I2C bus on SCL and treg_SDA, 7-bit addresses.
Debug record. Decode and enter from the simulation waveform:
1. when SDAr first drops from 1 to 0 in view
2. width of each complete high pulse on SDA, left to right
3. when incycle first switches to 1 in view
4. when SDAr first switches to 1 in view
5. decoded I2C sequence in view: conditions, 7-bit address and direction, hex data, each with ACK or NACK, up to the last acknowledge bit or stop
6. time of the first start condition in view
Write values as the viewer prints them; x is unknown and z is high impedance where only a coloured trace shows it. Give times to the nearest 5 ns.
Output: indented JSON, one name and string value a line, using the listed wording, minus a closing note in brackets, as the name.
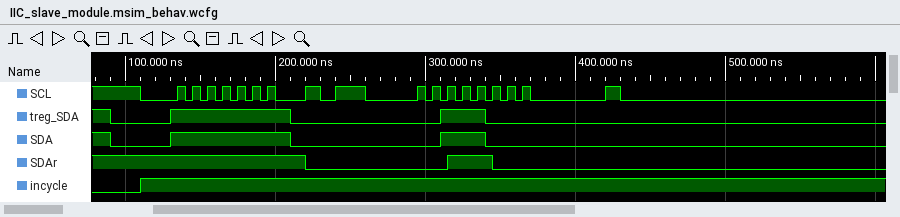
{
  "when SDAr first drops from 1 to 0 in view": "220 ns",
  "width of each complete high pulse on SDA, left to right": "80 ns, 30 ns",
  "when incycle first switches to 1 in view": "110 ns",
  "when SDAr first switches to 1 in view": "315 ns",
  "decoded I2C sequence in view: conditions, 7-bit address and direction, hex data, each with ACK or NACK, up to the last acknowledge bit or stop": "start, address 7F write ACK, 38 ACK",
  "time of the first start condition in view": "90 ns"
}
